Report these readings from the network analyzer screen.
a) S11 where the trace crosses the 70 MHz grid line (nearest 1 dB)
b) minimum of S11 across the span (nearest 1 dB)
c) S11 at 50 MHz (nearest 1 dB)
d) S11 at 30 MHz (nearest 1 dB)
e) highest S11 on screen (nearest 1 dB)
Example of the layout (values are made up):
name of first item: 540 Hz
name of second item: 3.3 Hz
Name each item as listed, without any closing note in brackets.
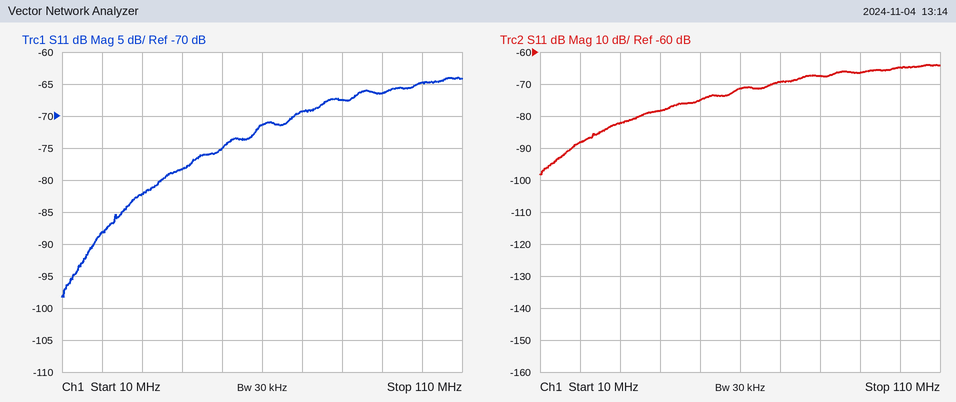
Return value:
S11 where the trace crosses the 70 MHz grid line: -69 dB
minimum of S11 across the span: -98 dB
S11 at 50 MHz: -75 dB
S11 at 30 MHz: -82 dB
highest S11 on screen: -64 dB
